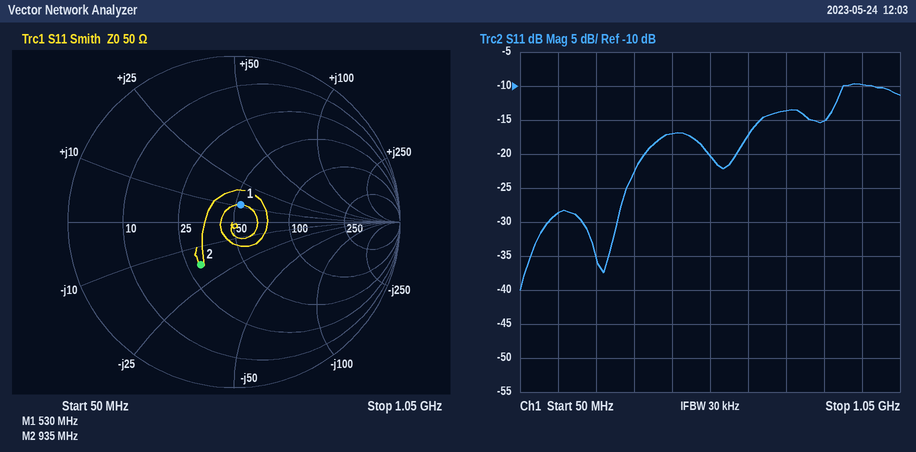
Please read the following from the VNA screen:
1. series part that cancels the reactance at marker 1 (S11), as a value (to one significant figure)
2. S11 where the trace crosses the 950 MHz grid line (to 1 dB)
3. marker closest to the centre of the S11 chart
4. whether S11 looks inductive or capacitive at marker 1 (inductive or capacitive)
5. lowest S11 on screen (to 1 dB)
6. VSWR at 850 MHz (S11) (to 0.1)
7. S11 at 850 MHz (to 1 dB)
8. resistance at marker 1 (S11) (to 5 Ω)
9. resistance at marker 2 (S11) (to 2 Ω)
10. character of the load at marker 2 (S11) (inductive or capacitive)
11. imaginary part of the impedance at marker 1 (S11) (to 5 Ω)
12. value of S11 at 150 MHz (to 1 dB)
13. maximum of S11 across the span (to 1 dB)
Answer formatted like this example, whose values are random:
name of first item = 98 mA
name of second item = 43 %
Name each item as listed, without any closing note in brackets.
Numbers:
series part that cancels the reactance at marker 1 (S11), as a value = 30 pF
S11 where the trace crosses the 950 MHz grid line = -10 dB
marker closest to the centre of the S11 chart = marker 1
whether S11 looks inductive or capacitive at marker 1 = inductive
lowest S11 on screen = -40 dB
VSWR at 850 MHz (S11) = 1.4
S11 at 850 MHz = -15 dB
resistance at marker 1 (S11) = 55 Ω
resistance at marker 2 (S11) = 30 Ω
character of the load at marker 2 (S11) = capacitive
imaginary part of the impedance at marker 1 (S11) = +10 Ω
value of S11 at 150 MHz = -29 dB
maximum of S11 across the span = -10 dB
